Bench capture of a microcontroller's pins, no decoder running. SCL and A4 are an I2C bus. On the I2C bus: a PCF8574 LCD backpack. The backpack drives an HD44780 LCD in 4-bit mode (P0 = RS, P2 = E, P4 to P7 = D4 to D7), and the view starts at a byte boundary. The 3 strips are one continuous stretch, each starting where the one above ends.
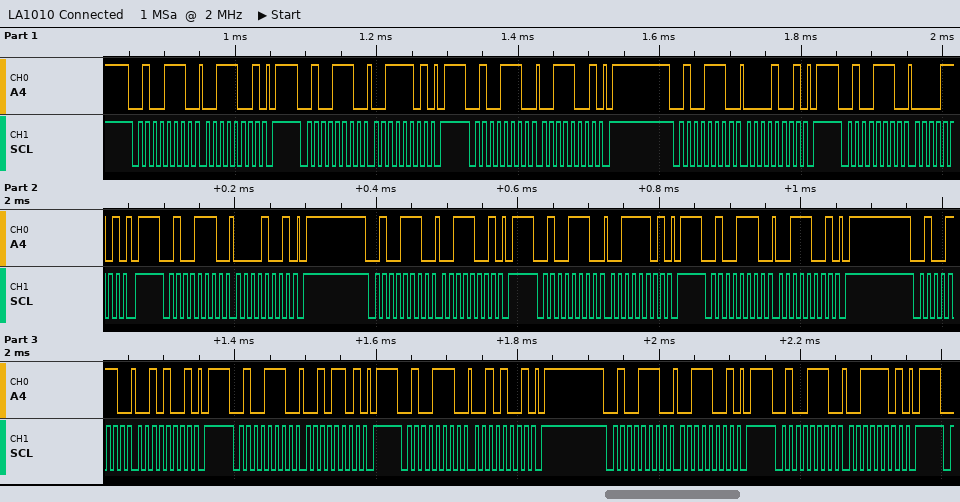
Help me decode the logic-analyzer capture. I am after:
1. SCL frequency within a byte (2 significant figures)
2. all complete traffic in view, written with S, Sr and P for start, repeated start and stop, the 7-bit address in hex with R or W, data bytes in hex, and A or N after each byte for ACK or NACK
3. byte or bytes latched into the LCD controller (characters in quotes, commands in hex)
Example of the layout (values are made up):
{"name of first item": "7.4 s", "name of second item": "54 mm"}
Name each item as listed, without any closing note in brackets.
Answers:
{"SCL frequency within a byte": "100 kHz", "all complete traffic in view, written with S, Sr and P for start, repeated start and stop, the 7-bit address in hex with R or W, data bytes in hex, and A or N after each byte for ACK or NACK": "S 27W A 39 A P S 27W A 3D A P S 27W A 39 A P S 27W A 09 A P S 27W A 0D A P S 27W A 09 A P S 27W A 39 A P S 27W A 3D A P S 27W A 39 A P S 27W A 29 A P S 27W A 2D A P S 27W A 29 A P S 27W A 39 A P S 27W A 3D A P", "byte or bytes latched into the LCD controller": "'0' '2'"}
